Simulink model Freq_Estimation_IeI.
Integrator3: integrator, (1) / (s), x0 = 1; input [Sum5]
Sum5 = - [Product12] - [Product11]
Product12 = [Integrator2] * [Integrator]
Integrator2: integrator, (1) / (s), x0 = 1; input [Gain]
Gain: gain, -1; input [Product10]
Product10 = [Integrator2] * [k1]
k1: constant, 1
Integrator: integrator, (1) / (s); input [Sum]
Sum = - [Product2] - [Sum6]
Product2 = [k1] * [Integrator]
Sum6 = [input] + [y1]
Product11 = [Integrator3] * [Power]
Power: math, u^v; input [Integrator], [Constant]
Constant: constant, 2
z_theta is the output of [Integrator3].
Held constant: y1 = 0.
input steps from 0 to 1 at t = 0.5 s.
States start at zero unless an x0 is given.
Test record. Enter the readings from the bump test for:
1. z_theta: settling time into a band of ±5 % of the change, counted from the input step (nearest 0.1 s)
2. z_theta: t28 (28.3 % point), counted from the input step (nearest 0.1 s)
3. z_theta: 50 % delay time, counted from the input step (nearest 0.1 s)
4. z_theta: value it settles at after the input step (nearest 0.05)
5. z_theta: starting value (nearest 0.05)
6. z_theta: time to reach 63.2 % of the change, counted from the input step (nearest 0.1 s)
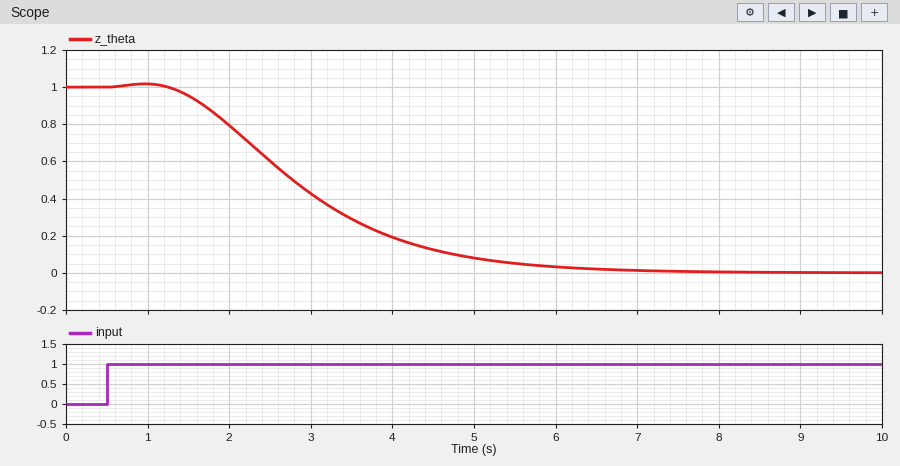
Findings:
5.0 s
1.7 s
2.3 s
0.00
1.00
2.7 s
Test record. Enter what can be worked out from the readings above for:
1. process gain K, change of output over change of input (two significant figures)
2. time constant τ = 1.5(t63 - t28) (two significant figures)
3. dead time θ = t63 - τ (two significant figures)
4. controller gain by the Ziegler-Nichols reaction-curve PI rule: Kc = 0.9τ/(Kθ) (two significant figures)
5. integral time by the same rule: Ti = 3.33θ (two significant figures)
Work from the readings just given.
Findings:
-1.0
1.5 s
1.2 s
-1.1
4.0 s
